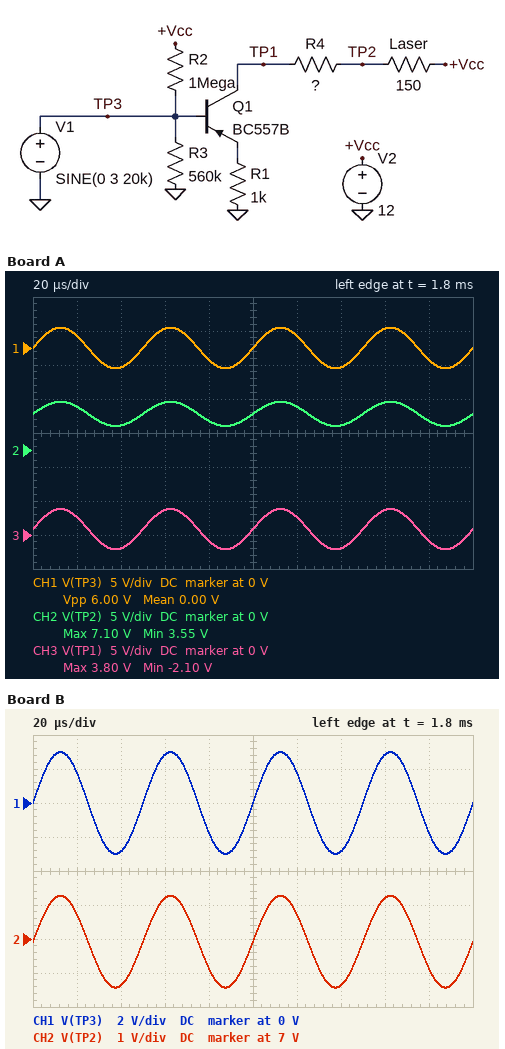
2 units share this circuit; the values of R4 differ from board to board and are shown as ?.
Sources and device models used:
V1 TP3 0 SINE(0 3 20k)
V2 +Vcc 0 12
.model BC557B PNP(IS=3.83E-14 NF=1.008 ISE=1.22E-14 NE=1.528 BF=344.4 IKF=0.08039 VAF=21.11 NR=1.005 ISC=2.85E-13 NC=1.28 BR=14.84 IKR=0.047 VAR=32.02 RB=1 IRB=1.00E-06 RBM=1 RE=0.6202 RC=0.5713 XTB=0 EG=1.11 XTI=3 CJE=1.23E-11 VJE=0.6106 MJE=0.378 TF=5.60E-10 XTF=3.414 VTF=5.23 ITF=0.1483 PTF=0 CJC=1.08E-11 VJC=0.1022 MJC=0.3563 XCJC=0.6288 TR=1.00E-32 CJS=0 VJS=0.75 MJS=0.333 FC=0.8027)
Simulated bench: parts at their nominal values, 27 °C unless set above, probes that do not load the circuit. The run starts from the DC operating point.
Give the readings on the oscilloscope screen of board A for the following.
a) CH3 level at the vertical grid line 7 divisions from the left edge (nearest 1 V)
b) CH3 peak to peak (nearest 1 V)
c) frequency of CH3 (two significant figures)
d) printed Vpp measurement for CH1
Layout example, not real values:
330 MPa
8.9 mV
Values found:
-2 V
6 V
20 kHz
6.00 V
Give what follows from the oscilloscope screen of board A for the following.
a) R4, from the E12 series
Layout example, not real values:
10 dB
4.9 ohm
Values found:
100 Ω
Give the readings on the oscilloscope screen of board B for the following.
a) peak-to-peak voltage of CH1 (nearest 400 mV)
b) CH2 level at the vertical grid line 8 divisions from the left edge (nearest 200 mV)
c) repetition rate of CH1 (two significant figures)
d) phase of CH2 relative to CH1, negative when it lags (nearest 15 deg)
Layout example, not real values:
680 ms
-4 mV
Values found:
6.0 V
8.2 V
20 kHz
0 deg
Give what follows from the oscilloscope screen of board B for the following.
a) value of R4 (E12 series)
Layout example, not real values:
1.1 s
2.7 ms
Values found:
180 Ω
